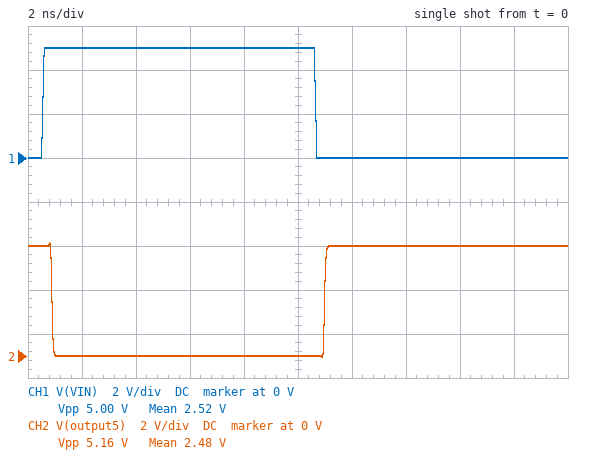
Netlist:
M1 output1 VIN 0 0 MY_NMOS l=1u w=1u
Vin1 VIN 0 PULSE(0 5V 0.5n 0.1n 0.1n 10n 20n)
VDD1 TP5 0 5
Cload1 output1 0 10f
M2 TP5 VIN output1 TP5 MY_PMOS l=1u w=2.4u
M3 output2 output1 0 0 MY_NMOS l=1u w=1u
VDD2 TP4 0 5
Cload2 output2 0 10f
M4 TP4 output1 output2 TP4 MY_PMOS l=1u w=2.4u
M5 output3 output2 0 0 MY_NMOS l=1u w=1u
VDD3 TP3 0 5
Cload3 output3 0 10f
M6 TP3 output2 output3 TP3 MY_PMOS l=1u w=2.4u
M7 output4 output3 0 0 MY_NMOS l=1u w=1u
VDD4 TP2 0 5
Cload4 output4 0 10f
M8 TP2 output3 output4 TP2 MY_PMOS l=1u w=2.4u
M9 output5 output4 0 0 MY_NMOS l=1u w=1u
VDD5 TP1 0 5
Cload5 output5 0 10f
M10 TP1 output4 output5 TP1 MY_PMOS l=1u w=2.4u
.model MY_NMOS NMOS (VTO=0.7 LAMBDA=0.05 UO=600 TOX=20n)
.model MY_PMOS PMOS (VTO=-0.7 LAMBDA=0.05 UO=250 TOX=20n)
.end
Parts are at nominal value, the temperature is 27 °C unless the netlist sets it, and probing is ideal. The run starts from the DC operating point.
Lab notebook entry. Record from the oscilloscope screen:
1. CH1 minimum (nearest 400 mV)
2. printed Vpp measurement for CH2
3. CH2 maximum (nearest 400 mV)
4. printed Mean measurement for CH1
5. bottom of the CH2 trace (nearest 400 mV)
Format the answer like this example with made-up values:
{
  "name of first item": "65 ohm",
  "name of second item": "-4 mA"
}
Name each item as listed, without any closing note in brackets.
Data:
{
  "CH1 minimum": "0 V",
  "printed Vpp measurement for CH2": "5.16 V",
  "CH2 maximum": "5.2 V",
  "printed Mean measurement for CH1": "2.52 V",
  "bottom of the CH2 trace": "0 V"
}
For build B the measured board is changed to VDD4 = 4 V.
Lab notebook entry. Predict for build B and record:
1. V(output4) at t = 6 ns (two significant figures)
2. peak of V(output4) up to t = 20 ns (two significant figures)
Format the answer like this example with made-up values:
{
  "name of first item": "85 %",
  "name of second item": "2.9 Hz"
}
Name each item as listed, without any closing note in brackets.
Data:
{
  "V(output4) at t = 6 ns": "4.0 V",
  "peak of V(output4) up to t = 20 ns": "4.1 V"
}
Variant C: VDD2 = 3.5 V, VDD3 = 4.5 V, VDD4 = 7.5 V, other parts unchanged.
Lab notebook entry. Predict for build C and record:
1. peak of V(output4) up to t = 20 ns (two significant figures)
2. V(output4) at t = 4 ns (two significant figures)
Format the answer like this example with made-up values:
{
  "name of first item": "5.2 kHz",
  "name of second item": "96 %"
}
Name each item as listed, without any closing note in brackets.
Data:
{
  "peak of V(output4) up to t = 20 ns": "7.6 V",
  "V(output4) at t = 4 ns": "7.5 V"
}
